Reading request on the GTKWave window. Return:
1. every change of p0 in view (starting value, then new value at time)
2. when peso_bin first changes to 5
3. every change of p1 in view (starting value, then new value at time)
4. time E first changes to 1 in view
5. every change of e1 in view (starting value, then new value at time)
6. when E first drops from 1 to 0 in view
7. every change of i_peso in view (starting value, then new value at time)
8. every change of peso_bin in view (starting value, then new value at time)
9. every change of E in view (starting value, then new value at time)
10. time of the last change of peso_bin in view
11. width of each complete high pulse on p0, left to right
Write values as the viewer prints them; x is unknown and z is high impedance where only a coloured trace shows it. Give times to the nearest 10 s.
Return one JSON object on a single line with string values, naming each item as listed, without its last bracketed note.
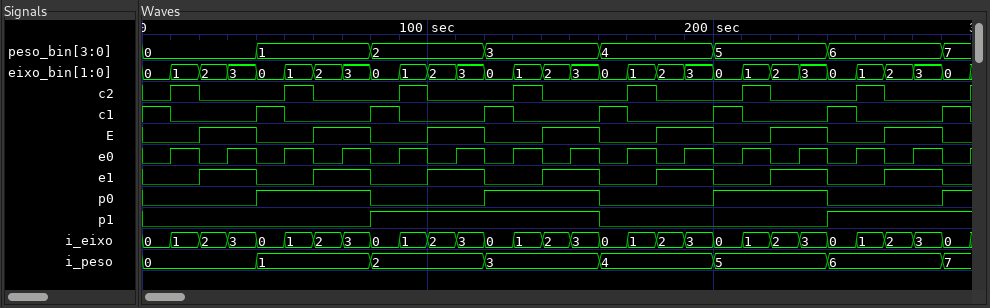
{"every change of p0 in view": "0, 1 at 40 s, 0 at 80 s, 1 at 120 s, 0 at 160 s, 1 at 200 s, 0 at 240 s, 1 at 280 s", "when peso_bin first changes to 5": "200 s", "every change of p1 in view": "0, 1 at 80 s, 0 at 160 s, 1 at 240 s", "time E first changes to 1 in view": "20 s", "every change of e1 in view": "0, 1 at 20 s, 0 at 40 s, 1 at 60 s, 0 at 80 s, 1 at 100 s, 0 at 120 s, 1 at 140 s, 0 at 160 s, 1 at 180 s, 0 at 200 s, 1 at 220 s, 0 at 240 s, 1 at 260 s, 0 at 280 s", "when E first drops from 1 to 0 in view": "40 s", "every change of i_peso in view": "0, 1 at 40 s, 2 at 80 s, 3 at 120 s, 4 at 160 s, 5 at 200 s, 6 at 240 s, 7 at 280 s", "every change of peso_bin in view": "0, 1 at 40 s, 2 at 80 s, 3 at 120 s, 4 at 160 s, 5 at 200 s, 6 at 240 s, 7 at 280 s", "every change of E in view": "0, 1 at 20 s, 0 at 40 s, 1 at 60 s, 0 at 80 s, 1 at 100 s, 0 at 120 s, 1 at 140 s, 0 at 160 s, 1 at 180 s, 0 at 200 s, 1 at 220 s, 0 at 240 s, 1 at 260 s, 0 at 280 s", "time of the last change of peso_bin in view": "280 s", "width of each complete high pulse on p0, left to right": "40 s, 40 s, 40 s"}
